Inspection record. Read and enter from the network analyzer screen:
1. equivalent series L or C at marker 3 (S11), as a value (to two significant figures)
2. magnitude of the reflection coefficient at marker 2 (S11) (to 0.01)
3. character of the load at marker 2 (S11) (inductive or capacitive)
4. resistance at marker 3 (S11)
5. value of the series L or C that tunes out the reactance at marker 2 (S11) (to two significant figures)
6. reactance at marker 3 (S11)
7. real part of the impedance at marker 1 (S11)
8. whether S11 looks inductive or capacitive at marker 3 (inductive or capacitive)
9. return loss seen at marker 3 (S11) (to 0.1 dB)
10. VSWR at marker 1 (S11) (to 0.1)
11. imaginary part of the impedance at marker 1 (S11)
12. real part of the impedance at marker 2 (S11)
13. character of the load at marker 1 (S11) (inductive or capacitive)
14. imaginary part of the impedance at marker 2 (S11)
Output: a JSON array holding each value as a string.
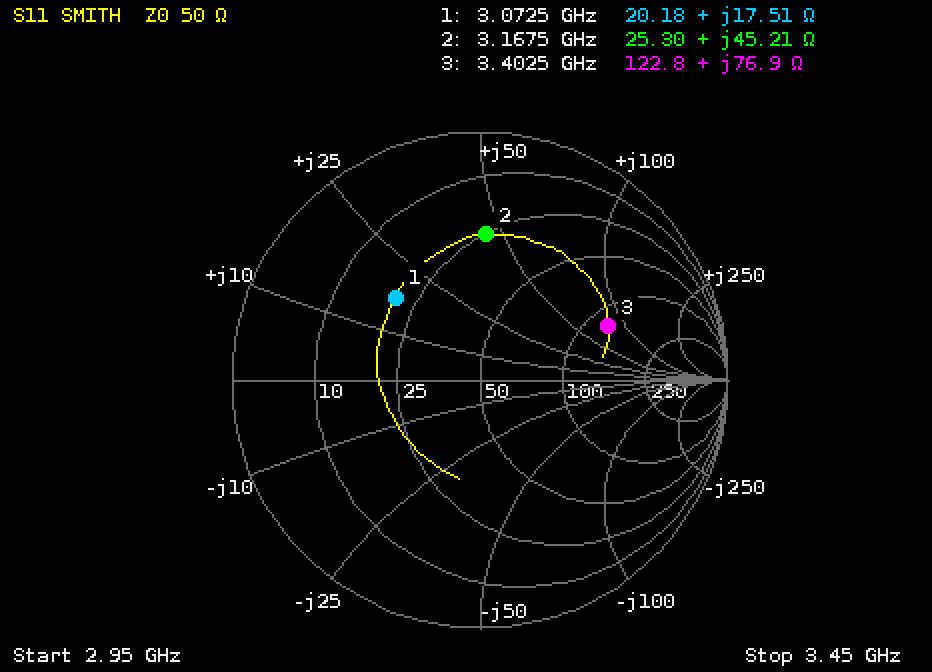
["3.6 nH", "0.59", "inductive", "122.8 Ω", "1.1 pF", "+76.9 Ω", "20.18 Ω", "inductive", "5.0 dB", "2.8", "+17.51 Ω", "25.30 Ω", "inductive", "+45.21 Ω"]
